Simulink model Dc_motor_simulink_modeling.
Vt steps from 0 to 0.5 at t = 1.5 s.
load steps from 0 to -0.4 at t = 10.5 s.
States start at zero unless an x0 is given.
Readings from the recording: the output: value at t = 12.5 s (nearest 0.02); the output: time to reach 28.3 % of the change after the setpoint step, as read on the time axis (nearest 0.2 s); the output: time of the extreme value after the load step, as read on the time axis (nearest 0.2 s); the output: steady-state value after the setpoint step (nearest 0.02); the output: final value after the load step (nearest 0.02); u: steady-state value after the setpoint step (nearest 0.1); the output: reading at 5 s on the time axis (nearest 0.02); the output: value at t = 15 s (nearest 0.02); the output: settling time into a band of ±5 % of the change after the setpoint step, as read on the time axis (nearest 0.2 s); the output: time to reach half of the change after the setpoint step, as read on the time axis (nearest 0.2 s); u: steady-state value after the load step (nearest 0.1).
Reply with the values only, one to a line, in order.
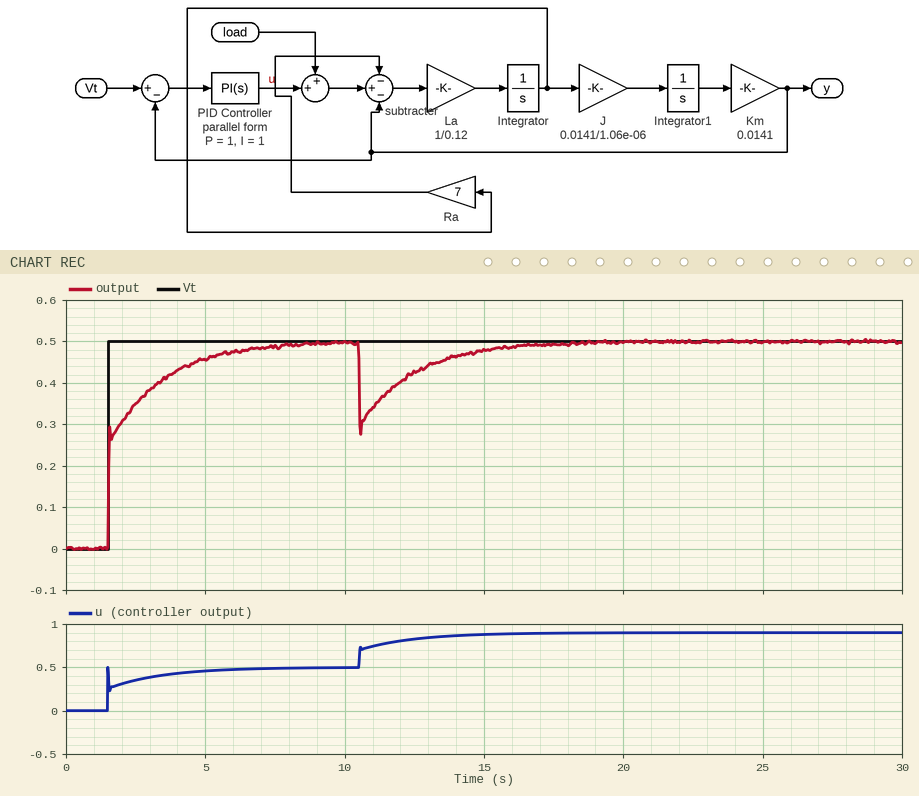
0.42
1.6 s
10.6 s
0.50
0.50
0.5
0.46
0.48
6.0 s
1.6 s
0.9
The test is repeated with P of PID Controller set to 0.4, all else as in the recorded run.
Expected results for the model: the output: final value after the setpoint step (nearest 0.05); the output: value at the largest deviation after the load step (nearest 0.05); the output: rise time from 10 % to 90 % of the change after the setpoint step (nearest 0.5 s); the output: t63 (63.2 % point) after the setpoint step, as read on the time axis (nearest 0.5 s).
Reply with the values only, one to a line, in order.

0.50
0.20
2.5 s
2.5 s
